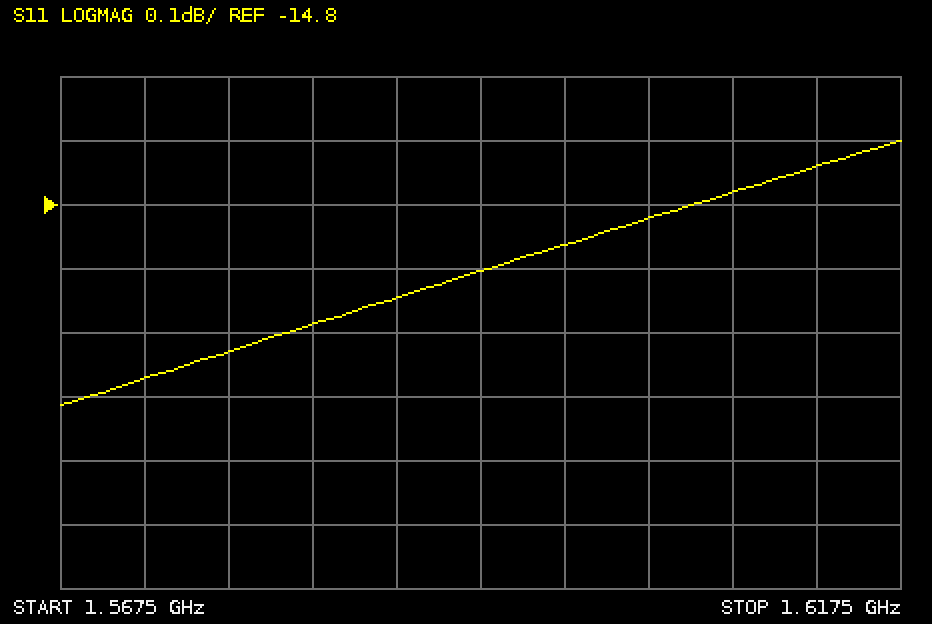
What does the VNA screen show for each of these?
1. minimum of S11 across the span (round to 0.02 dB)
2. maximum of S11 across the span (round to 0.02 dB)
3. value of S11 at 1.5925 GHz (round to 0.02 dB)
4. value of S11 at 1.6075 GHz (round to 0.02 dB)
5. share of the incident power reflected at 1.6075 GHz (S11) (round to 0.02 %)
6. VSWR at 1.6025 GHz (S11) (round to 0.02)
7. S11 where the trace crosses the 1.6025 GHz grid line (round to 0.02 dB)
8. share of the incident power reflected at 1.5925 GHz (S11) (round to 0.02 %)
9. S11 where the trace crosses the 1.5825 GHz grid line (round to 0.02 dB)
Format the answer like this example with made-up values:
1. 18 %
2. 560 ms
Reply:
1. -15.12 dB
2. -14.70 dB
3. -14.90 dB
4. -14.78 dB
5. 3.32 %
6. 1.44
7. -14.82 dB
8. 3.24 %
9. -14.98 dB
